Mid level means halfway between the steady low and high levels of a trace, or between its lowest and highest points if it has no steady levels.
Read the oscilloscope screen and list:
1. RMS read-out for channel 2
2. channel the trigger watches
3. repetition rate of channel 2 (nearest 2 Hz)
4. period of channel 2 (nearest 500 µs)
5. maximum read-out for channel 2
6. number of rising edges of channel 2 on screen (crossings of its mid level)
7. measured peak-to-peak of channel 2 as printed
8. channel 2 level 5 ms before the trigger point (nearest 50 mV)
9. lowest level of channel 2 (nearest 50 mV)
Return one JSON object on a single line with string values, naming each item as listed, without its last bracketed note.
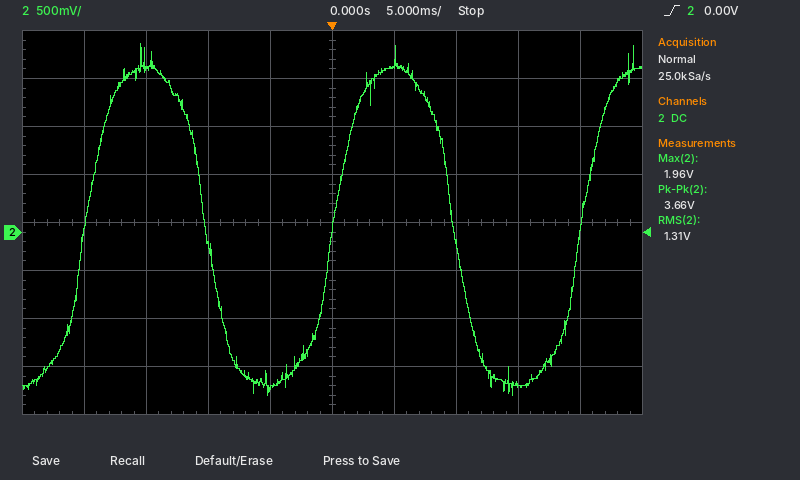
{"RMS read-out for channel 2": "1.31 V", "channel the trigger watches": "channel 2", "repetition rate of channel 2": "50 Hz", "period of channel 2": "20.0 ms", "maximum read-out for channel 2": "1.96 V", "number of rising edges of channel 2 on screen": "3", "measured peak-to-peak of channel 2 as printed": "3.66 V", "channel 2 level 5 ms before the trigger point": "-1.65 V", "lowest level of channel 2": "-1.70 V"}
